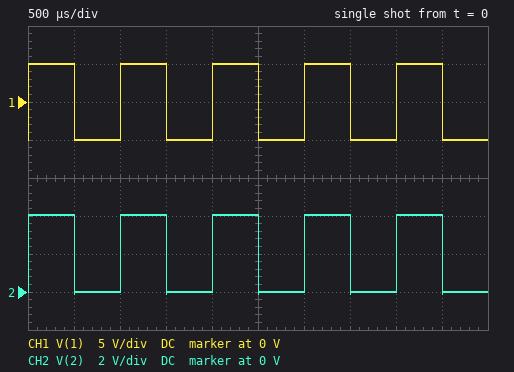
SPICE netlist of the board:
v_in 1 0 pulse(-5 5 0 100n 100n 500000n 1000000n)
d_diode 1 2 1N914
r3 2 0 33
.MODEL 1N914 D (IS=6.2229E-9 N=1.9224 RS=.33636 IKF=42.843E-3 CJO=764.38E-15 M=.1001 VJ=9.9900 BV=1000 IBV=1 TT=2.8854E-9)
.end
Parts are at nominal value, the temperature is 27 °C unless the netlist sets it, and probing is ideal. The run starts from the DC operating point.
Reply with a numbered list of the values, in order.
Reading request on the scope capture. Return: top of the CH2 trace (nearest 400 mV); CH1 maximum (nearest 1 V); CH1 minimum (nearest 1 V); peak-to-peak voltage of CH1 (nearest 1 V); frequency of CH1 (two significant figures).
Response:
1. 4.0 V
2. 5 V
3. -5 V
4. 10 V
5. 1.0 kHz
